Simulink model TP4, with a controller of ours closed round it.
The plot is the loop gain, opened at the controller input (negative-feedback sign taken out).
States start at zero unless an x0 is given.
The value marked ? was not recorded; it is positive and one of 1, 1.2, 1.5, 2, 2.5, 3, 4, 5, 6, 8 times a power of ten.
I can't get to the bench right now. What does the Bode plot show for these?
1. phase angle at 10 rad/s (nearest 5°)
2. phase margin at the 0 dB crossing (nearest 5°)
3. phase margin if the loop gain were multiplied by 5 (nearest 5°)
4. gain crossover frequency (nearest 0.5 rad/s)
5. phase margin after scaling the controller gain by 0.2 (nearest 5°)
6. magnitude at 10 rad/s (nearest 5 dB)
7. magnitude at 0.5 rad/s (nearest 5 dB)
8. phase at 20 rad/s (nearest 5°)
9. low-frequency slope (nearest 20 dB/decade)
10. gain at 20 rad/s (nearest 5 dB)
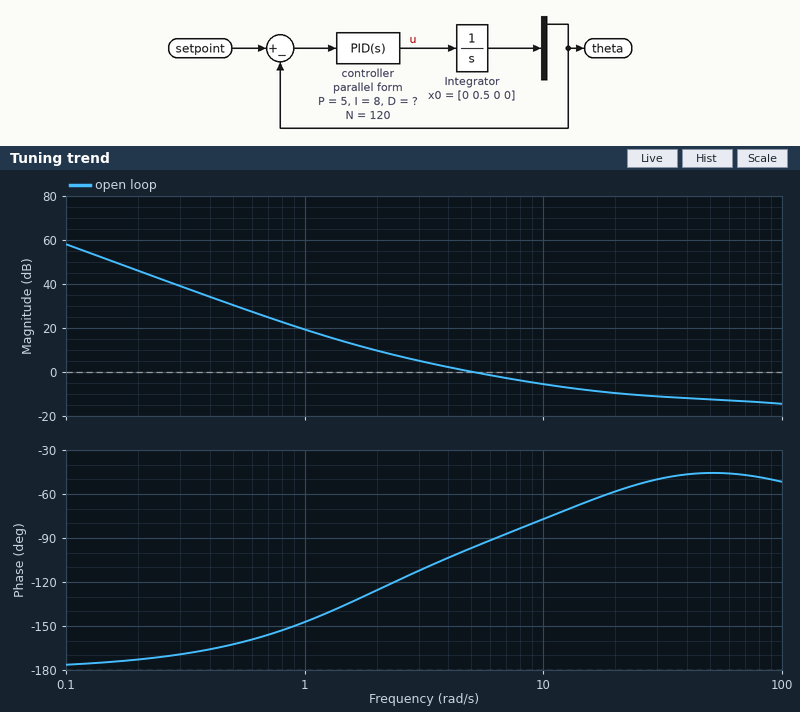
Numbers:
-75°
85°
130°
5.0 rad/s
45°
-5 dB
30 dB
-60°
-40 dB/decade
-10 dB
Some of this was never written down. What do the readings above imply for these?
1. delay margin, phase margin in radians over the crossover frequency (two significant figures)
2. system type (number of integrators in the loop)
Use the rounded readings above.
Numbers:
0.30 s
2
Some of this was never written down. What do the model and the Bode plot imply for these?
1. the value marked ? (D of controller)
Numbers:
0.2
